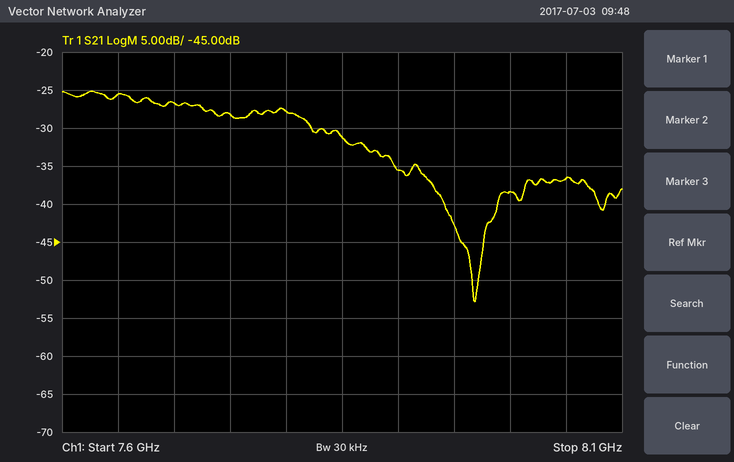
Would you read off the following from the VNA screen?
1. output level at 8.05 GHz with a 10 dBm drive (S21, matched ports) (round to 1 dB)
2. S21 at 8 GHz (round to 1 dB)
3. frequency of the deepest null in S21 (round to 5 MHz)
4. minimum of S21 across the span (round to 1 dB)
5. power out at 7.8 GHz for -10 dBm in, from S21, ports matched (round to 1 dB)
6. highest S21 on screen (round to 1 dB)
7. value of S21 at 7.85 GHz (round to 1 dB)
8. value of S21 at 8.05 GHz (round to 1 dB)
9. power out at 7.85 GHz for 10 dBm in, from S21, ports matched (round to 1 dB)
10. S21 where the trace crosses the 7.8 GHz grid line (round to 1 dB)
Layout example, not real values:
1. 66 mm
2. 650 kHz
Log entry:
1. -27 dBm
2. -38 dB
3. 7.970 GHz
4. -53 dB
5. -38 dBm
6. -25 dB
7. -31 dB
8. -37 dB
9. -21 dBm
10. -28 dB
